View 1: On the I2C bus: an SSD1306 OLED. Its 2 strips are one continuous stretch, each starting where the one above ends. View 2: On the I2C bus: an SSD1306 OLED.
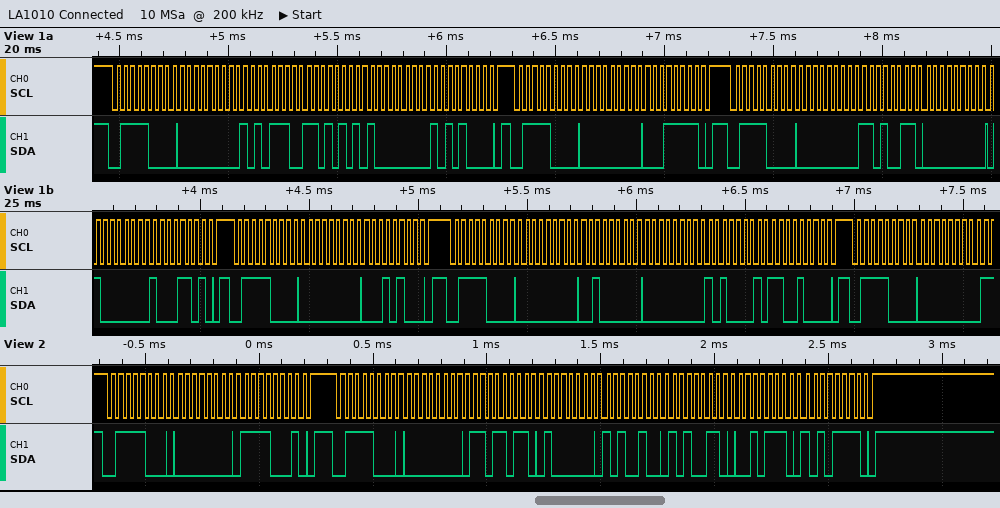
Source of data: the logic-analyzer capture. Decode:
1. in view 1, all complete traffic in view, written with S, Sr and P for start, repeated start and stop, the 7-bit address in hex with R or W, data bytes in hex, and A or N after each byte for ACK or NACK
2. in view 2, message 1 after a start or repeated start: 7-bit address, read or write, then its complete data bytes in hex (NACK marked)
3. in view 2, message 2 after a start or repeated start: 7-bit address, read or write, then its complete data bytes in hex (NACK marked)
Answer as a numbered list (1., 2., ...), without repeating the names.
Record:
1. S 3CW A 00 A AE A D5 A 80 A A8 A P S 3CW A 00 A 1F A P S 3CW A 00 A D3 A 00 A 40 A 8D A P S 3CW A 00 A 14 A P S 3CW A 00 A 20 A 00 A A1 A C8 A P S 3CW A 00 A
2. 0x3C write: 00 F1
3. 0x3C write: 00 DB 40 A4 A6 2E AF
